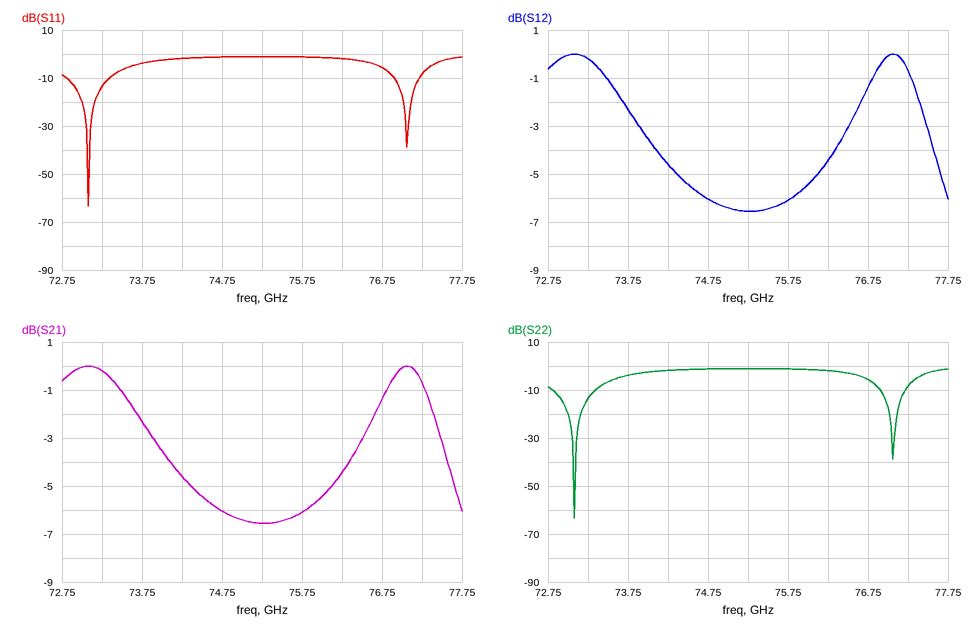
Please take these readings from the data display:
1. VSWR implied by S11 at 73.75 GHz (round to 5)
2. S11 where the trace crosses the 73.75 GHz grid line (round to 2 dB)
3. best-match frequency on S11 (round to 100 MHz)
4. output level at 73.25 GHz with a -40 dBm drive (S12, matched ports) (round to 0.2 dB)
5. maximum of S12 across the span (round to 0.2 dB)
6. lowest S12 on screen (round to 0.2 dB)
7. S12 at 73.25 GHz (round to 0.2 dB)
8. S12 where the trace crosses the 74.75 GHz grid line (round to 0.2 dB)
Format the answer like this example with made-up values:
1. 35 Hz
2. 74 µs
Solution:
1. 5
2. -4 dB
3. 73.1 GHz
4. -40.2 dBm
5. 0.0 dB
6. -6.6 dB
7. -0.2 dB
8. -6.0 dB
